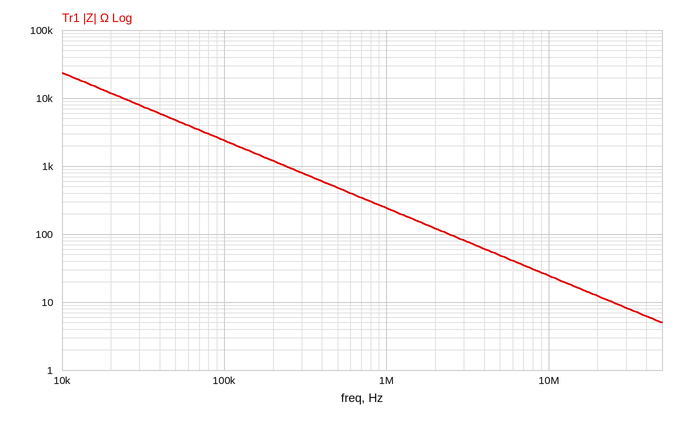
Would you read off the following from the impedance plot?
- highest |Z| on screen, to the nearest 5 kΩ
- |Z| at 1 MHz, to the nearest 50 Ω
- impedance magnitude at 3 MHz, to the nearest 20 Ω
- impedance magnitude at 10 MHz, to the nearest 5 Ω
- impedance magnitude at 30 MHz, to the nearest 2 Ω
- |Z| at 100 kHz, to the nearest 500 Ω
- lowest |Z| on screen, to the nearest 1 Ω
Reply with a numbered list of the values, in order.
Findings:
1. 25 kΩ
2. 250 Ω
3. 80 Ω
4. 25 Ω
5. 8 Ω
6. 2.5 kΩ
7. 5 Ω
